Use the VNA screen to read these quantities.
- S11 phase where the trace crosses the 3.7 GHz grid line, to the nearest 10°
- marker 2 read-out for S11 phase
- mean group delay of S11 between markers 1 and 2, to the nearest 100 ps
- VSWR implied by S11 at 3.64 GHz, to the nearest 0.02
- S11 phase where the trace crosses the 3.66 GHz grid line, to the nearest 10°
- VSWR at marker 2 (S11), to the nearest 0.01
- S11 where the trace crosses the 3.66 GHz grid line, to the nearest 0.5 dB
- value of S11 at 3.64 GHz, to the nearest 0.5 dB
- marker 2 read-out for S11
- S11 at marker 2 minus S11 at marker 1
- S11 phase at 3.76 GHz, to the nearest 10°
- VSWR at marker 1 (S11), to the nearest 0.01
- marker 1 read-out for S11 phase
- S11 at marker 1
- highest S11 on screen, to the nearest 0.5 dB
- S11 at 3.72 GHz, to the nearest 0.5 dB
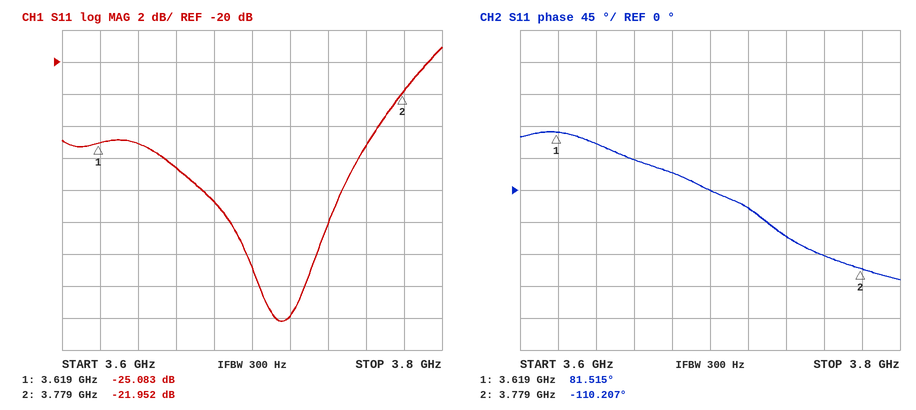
0°
-110.207°
3.3 ns
1.12
40°
1.17
-26.5 dB
-25.0 dB
-21.952 dB
3.131 dB
-90°
1.12
81.515°
-25.083 dB
-19.0 dB
-36.0 dB
